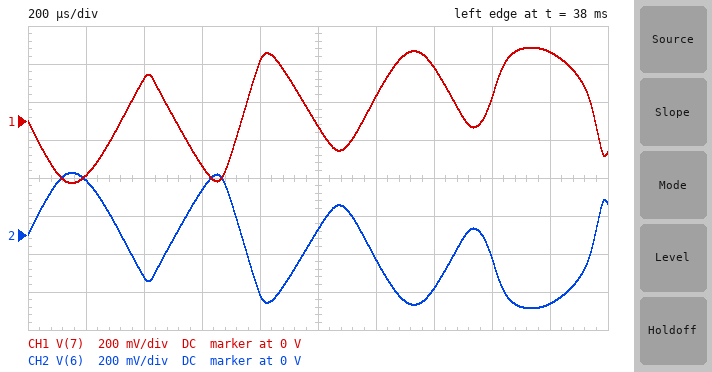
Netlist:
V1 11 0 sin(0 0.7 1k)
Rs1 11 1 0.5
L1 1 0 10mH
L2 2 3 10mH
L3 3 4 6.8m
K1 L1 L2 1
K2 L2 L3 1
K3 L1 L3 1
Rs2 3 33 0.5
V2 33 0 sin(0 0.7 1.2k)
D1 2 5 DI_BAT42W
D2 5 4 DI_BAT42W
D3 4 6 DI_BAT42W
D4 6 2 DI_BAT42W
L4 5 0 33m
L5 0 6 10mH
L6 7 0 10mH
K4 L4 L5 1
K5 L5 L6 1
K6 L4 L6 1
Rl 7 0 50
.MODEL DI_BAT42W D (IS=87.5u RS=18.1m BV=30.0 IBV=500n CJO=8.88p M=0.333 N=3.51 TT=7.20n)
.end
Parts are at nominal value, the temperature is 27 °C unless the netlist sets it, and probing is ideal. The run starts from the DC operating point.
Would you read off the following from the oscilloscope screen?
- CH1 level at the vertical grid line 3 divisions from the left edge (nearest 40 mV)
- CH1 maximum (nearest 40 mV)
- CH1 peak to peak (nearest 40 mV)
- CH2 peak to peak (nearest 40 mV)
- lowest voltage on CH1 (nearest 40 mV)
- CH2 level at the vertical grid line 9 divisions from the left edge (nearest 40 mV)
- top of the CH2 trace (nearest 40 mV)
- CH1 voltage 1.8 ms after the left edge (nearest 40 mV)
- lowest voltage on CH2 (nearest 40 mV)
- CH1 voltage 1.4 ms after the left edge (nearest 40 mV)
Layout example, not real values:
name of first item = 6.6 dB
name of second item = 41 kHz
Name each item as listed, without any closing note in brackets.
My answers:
CH1 level at the vertical grid line 3 divisions from the left edge = -240 mV
CH1 maximum = 400 mV
CH1 peak to peak = 720 mV
CH2 peak to peak = 720 mV
lowest voltage on CH1 = -320 mV
CH2 level at the vertical grid line 9 divisions from the left edge = -360 mV
top of the CH2 trace = 320 mV
CH1 voltage 1.8 ms after the left edge = 360 mV
lowest voltage on CH2 = -400 mV
CH1 voltage 1.4 ms after the left edge = 280 mV
